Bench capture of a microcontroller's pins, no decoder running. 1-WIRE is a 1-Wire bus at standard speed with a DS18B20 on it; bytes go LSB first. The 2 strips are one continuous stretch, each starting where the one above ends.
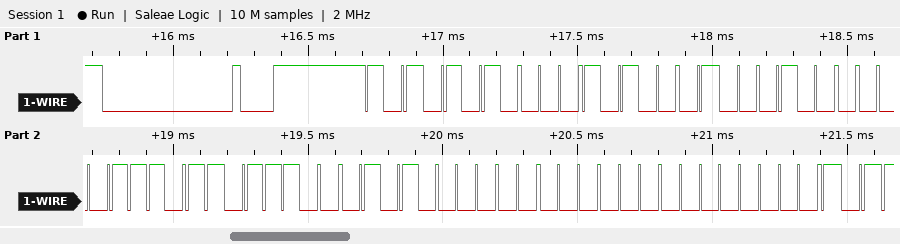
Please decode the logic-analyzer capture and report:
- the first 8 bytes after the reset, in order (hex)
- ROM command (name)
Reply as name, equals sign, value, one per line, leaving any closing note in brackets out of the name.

the first 8 bytes after the reset, in order = 55 28 22 70 3B 0A 00 00
ROM command = Match ROM
